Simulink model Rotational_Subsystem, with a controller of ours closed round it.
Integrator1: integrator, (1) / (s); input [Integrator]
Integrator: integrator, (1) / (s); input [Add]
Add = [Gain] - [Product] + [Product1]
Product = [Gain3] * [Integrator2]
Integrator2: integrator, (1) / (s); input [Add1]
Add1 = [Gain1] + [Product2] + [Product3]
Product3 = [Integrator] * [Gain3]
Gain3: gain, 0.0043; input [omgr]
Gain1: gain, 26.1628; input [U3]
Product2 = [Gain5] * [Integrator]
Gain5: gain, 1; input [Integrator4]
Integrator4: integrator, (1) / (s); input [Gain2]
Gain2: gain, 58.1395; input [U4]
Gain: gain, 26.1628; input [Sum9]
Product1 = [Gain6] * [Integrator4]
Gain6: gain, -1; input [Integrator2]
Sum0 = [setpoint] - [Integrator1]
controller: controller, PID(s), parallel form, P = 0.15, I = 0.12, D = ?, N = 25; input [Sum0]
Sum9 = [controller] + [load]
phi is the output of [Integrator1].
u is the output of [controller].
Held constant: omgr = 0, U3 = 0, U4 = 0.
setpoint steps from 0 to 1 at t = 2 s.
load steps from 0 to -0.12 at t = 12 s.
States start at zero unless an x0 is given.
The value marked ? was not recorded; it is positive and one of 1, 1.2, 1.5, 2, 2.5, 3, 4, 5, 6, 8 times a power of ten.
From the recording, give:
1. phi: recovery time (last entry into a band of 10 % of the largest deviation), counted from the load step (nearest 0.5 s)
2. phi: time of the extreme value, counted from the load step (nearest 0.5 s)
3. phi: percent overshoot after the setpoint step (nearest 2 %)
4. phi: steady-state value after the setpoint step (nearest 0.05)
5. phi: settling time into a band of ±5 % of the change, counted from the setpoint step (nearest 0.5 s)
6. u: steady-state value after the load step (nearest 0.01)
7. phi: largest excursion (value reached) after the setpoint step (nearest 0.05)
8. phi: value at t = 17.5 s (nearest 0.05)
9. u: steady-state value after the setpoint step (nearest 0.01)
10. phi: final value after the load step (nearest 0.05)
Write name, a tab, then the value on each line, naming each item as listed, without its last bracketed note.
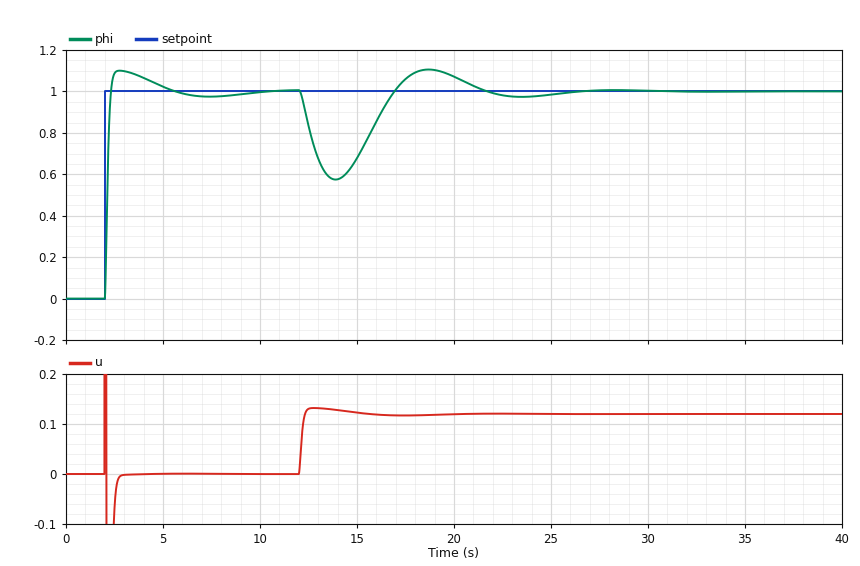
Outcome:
phi: recovery time (last entry into a band of 10 % of the largest deviation), counted from the load step	8.5 s
phi: time of the extreme value, counted from the load step	2.0 s
phi: percent overshoot after the setpoint step	10 %
phi: steady-state value after the setpoint step	1.00
phi: settling time into a band of ±5 % of the change, counted from the setpoint step	2.5 s
u: steady-state value after the load step	0.12
phi: largest excursion (value reached) after the setpoint step	1.10
phi: value at t = 17.5 s	1.05
u: steady-state value after the setpoint step	0.00
phi: final value after the load step	1.00
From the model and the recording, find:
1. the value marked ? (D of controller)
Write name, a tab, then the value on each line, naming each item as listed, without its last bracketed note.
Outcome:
the value marked ?	0.25
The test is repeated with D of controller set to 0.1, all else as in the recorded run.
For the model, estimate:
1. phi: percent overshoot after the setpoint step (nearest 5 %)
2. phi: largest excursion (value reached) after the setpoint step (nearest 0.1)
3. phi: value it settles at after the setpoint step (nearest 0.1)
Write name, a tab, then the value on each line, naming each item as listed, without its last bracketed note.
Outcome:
phi: percent overshoot after the setpoint step	35 %
phi: largest excursion (value reached) after the setpoint step	1.4
phi: value it settles at after the setpoint step	1.0
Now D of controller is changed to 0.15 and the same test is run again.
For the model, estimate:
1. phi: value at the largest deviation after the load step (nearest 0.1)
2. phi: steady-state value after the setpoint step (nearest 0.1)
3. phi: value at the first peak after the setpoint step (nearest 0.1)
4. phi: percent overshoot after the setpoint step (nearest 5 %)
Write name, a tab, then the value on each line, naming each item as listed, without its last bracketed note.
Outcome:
phi: value at the largest deviation after the load step	0.5
phi: steady-state value after the setpoint step	1.0
phi: value at the first peak after the setpoint step	1.2
phi: percent overshoot after the setpoint step	20 %
